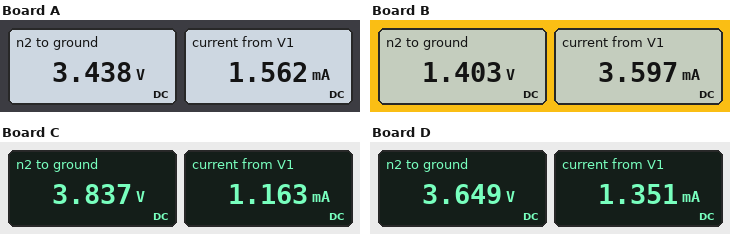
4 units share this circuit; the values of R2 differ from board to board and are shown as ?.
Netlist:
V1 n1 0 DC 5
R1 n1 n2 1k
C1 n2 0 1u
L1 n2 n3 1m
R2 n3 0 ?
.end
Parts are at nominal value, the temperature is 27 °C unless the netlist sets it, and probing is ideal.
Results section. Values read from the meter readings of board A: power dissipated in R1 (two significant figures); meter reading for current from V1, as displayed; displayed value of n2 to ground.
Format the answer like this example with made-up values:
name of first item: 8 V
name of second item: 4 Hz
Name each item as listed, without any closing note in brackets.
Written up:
power dissipated in R1: 2.4 mW
meter reading for current from V1, as displayed: 1.562 mA
displayed value of n2 to ground: 3.438 V
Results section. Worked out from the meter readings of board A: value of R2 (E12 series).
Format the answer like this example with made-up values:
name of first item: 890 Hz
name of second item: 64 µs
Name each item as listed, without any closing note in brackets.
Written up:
value of R2: 2.2 kΩ
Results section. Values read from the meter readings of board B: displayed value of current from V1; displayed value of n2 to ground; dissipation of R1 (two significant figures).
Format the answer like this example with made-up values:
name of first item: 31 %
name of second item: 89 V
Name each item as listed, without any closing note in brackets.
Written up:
displayed value of current from V1: 3.597 mA
displayed value of n2 to ground: 1.403 V
dissipation of R1: 13 mW
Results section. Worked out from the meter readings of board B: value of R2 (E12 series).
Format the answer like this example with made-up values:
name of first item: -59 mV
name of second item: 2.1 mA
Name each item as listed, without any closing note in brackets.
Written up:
value of R2: 390 Ω
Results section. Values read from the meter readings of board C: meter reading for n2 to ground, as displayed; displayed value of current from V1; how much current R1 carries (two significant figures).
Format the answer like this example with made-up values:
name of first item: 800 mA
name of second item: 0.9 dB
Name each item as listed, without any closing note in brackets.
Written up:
meter reading for n2 to ground, as displayed: 3.837 V
displayed value of current from V1: 1.163 mA
how much current R1 carries: 1.2 mA
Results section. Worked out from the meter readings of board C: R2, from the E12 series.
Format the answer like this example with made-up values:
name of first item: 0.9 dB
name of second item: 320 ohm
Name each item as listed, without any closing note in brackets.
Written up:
R2, from the E12 series: 3.3 kΩ
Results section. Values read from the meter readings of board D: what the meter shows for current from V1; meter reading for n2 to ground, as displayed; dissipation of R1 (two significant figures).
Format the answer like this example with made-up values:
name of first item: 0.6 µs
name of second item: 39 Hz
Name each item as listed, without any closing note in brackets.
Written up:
what the meter shows for current from V1: 1.351 mA
meter reading for n2 to ground, as displayed: 3.649 V
dissipation of R1: 1.8 mW
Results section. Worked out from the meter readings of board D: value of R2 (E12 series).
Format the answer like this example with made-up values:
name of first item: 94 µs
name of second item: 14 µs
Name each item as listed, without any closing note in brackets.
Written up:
value of R2: 2.7 kΩ
